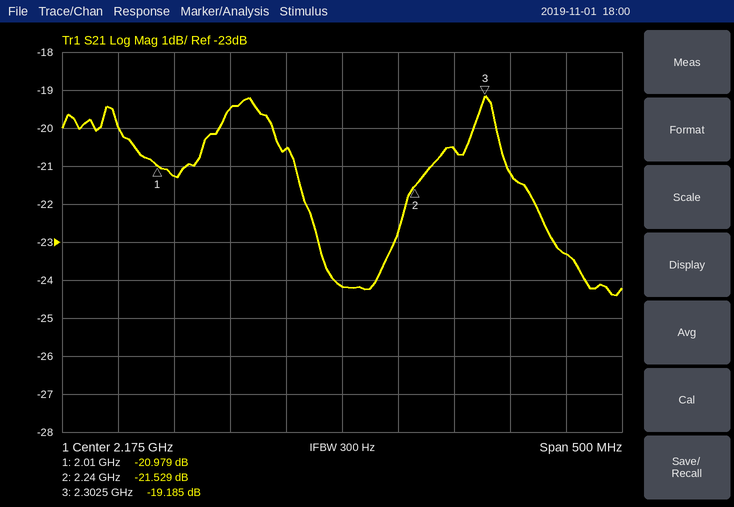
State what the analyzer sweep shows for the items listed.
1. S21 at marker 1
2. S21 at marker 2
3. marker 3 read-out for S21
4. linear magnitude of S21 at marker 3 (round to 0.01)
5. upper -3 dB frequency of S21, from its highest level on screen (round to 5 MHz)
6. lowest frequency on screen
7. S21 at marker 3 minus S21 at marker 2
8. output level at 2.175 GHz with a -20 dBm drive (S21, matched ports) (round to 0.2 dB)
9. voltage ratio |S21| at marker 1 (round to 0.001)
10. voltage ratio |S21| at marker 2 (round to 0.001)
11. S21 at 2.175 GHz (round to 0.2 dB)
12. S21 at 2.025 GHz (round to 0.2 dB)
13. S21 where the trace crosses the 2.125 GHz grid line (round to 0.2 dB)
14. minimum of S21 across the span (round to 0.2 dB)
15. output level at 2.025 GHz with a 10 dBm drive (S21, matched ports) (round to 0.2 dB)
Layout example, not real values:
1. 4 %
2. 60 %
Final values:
1. -20.979 dB
2. -21.529 dB
3. -19.185 dB
4. 0.11
5. 2.350 GHz
6. 1.925 GHz
7. 2.344 dB
8. -44.2 dBm
9. 0.089
10. 0.084
11. -24.2 dB
12. -21.2 dB
13. -20.6 dB
14. -24.4 dB
15. -11.2 dBm
